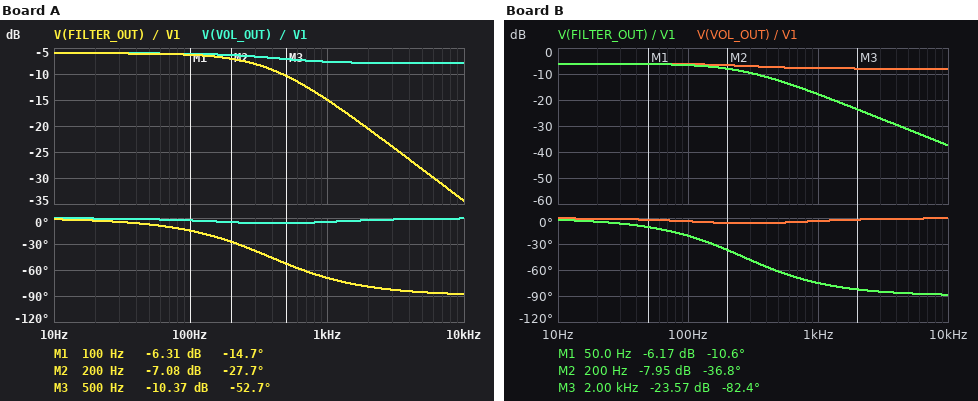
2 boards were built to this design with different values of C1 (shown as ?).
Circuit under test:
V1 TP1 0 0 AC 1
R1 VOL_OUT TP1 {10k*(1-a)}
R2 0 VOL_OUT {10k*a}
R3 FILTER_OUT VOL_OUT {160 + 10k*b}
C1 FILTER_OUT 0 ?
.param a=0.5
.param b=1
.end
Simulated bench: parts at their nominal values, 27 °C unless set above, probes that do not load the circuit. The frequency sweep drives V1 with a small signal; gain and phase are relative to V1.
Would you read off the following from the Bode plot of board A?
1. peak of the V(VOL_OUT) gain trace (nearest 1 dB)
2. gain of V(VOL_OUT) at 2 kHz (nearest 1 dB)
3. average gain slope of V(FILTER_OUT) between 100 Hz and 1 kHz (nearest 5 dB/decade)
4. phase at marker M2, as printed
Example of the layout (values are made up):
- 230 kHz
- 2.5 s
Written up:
- -6 dB
- -8 dB
- -10 dB/decade
- -27.7 deg
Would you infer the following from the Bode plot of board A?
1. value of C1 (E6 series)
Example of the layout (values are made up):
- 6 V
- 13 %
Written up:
- 33 nF
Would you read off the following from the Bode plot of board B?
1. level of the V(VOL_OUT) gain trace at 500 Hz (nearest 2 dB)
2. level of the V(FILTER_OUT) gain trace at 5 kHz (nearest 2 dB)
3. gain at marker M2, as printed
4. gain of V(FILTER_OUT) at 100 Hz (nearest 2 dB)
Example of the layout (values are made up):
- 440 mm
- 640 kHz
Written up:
- -8 dB
- -32 dB
- -7.95 dB
- -6 dB
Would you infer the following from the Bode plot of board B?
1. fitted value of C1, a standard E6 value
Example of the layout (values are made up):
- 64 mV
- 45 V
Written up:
- 47 nF
